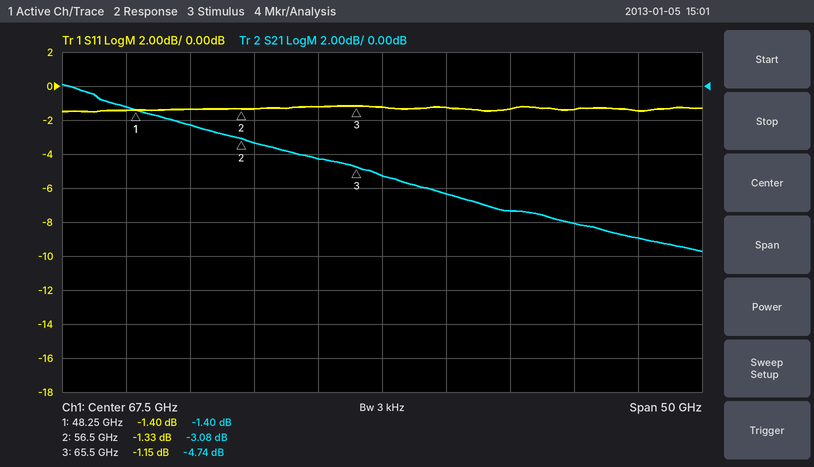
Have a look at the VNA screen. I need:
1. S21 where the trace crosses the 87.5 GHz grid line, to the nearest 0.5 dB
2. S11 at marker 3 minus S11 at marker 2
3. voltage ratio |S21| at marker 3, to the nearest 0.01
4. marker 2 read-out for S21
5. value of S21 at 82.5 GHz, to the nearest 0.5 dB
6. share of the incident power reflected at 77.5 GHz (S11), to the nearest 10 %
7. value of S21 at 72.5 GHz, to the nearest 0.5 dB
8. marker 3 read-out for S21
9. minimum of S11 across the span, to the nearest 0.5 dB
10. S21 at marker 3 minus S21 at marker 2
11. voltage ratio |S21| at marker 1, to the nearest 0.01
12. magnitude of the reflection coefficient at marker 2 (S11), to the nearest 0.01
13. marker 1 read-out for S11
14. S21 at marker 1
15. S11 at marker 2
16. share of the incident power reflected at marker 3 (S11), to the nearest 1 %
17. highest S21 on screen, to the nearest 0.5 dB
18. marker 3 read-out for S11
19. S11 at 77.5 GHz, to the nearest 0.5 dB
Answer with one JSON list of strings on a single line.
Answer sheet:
["-9.0 dB", "0.18 dB", "0.58", "-3.08 dB", "-8.0 dB", "70 %", "-6.5 dB", "-4.74 dB", "-1.5 dB", "-1.66 dB", "0.85", "0.86", "-1.40 dB", "-1.40 dB", "-1.33 dB", "77 %", "0.0 dB", "-1.15 dB", "-1.5 dB"]
